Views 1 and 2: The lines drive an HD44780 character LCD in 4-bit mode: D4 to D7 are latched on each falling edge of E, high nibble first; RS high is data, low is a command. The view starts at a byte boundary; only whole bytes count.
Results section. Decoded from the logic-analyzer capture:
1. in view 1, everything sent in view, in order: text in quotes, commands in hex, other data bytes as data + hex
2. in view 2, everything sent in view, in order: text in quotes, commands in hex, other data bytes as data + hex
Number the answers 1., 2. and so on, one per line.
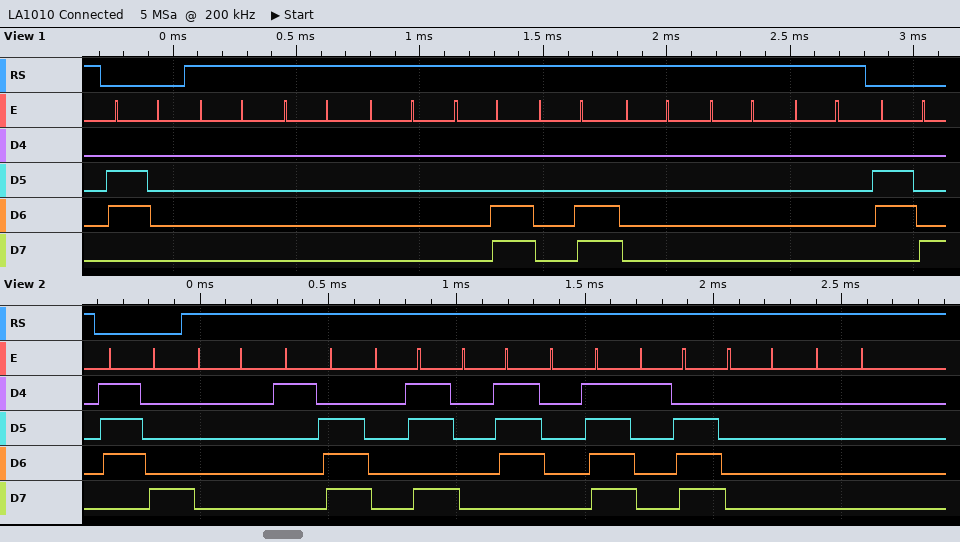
1. 0x60 data 00 00 00 0C 0C 00 00 00 0x68
2. 0x78 data 00 1E 0B 07 0F 1E 00 00
